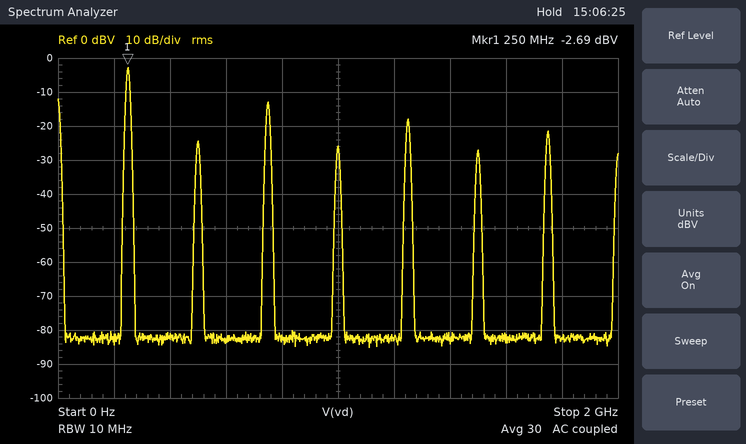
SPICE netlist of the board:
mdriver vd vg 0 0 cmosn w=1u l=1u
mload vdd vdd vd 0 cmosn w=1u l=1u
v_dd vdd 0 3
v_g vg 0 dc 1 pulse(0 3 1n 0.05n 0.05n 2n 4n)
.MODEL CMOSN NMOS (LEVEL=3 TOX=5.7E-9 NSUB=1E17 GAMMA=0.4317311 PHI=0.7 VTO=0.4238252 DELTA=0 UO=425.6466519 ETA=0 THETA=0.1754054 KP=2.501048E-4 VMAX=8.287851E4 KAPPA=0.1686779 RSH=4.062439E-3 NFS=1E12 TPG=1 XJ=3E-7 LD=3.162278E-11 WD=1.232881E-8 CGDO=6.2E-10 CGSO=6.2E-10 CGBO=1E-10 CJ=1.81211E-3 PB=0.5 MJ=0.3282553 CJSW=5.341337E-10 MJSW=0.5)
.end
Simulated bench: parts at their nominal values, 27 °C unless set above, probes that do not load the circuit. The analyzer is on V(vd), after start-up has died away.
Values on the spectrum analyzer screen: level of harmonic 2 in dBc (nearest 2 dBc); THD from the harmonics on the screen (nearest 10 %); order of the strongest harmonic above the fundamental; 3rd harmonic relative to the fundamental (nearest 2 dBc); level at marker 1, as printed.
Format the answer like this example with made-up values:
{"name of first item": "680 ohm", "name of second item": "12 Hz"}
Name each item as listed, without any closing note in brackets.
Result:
{"level of harmonic 2 in dBc": "-22 dBc", "THD from the harmonics on the screen": "40 %", "order of the strongest harmonic above the fundamental": "3", "3rd harmonic relative to the fundamental": "-10 dBc", "level at marker 1, as printed": "-2.69 dBV"}
